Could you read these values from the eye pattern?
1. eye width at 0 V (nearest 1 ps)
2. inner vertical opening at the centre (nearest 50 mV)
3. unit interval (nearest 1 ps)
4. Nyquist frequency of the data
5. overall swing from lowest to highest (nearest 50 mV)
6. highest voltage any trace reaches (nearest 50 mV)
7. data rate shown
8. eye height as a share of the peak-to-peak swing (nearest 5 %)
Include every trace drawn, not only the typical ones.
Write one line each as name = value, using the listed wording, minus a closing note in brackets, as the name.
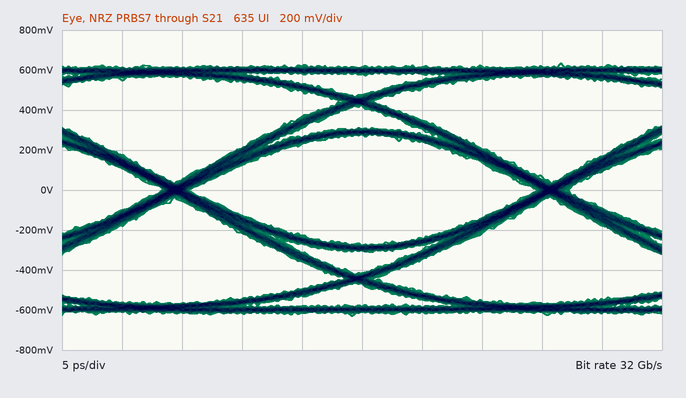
eye width at 0 V = 29 ps
inner vertical opening at the centre = 550 mV
unit interval = 31 ps
Nyquist frequency of the data = 16 GHz
overall swing from lowest to highest = 1.25 V
highest voltage any trace reaches = 650 mV
data rate shown = 32 Gb/s
eye height as a share of the peak-to-peak swing = 45 %
